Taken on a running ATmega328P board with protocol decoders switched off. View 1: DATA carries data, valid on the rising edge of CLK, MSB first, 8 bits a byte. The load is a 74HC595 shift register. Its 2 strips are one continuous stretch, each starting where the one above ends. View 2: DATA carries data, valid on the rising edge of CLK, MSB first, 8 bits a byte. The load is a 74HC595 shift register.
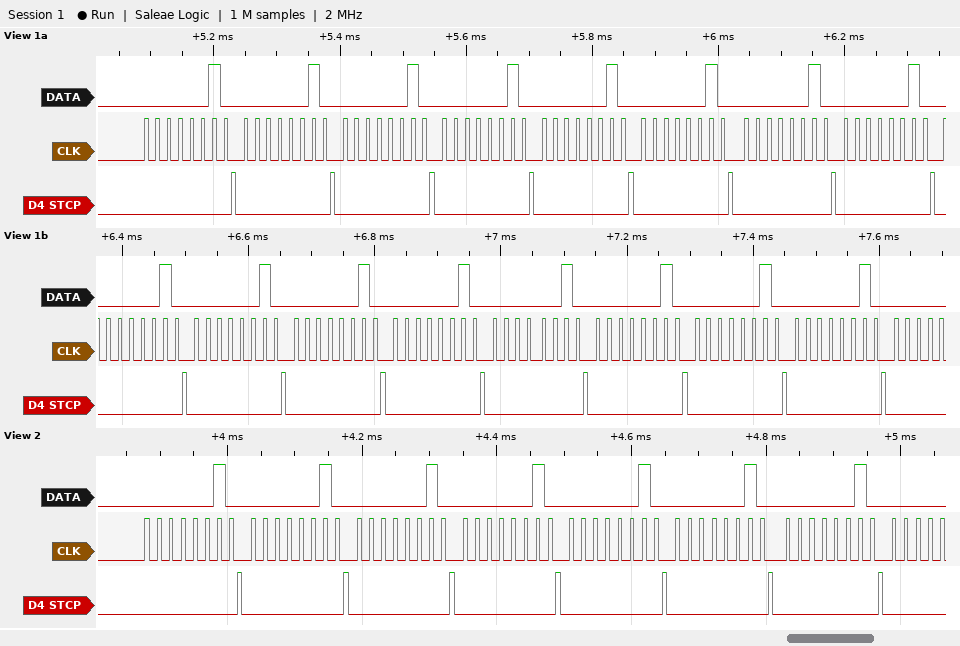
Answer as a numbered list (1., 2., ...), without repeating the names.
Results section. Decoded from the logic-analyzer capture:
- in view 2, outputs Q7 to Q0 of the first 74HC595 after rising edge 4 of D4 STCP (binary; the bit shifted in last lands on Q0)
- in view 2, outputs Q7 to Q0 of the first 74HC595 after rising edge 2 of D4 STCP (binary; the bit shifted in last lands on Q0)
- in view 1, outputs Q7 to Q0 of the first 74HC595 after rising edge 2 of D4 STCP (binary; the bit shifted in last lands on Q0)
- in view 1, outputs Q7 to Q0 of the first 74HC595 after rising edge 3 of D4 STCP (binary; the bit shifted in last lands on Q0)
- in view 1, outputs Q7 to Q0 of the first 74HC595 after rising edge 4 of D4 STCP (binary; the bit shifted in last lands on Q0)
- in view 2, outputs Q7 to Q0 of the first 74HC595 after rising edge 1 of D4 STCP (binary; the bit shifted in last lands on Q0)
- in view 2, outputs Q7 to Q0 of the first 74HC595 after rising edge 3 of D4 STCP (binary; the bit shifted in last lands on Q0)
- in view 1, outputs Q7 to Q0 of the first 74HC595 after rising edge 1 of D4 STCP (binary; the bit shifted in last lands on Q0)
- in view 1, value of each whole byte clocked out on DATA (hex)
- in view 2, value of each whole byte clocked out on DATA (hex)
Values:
1. 00000010
2. 00000010
3. 00000010
4. 00000010
5. 00000010
6. 00000010
7. 00000010
8. 00000010
9. 02 02 02 02 02 02 02 02 02 02 02 02 02 02 02 02
10. 02 02 02 02 02 02 02
